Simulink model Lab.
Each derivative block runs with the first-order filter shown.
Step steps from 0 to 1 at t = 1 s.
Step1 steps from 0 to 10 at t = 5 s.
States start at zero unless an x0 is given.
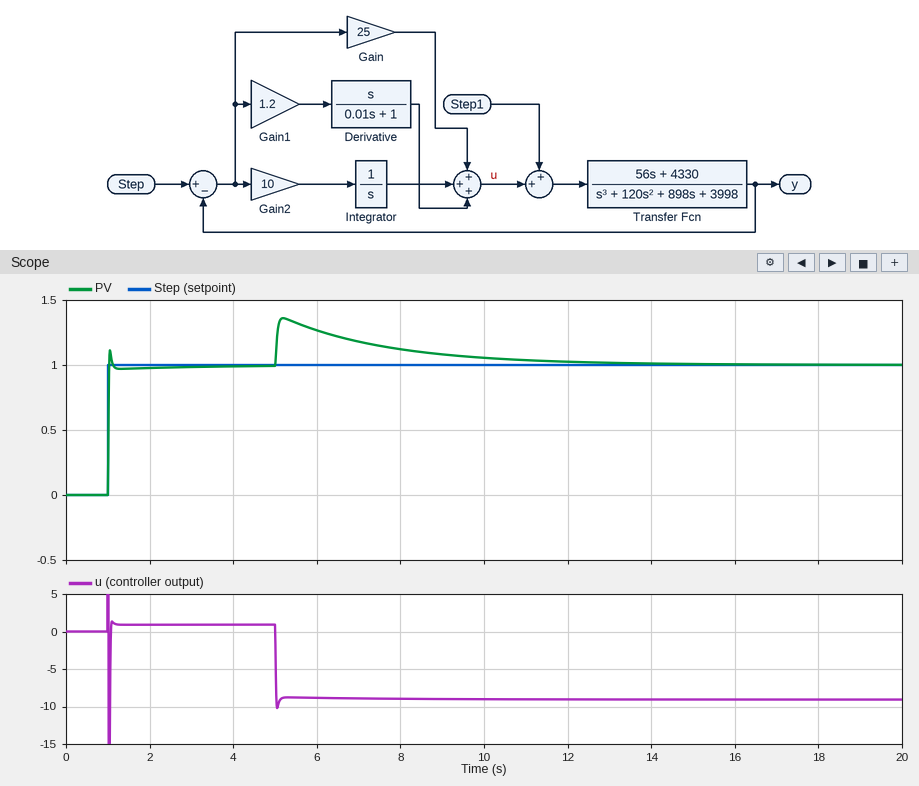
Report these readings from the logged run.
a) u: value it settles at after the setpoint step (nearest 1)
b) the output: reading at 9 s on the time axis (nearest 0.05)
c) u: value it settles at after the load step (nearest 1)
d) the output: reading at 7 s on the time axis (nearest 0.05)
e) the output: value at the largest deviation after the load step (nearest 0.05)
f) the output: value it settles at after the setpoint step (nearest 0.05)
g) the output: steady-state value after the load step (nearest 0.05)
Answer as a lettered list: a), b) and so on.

a) 1
b) 1.10
c) -9
d) 1.20
e) 1.35
f) 1.00
g) 1.00
